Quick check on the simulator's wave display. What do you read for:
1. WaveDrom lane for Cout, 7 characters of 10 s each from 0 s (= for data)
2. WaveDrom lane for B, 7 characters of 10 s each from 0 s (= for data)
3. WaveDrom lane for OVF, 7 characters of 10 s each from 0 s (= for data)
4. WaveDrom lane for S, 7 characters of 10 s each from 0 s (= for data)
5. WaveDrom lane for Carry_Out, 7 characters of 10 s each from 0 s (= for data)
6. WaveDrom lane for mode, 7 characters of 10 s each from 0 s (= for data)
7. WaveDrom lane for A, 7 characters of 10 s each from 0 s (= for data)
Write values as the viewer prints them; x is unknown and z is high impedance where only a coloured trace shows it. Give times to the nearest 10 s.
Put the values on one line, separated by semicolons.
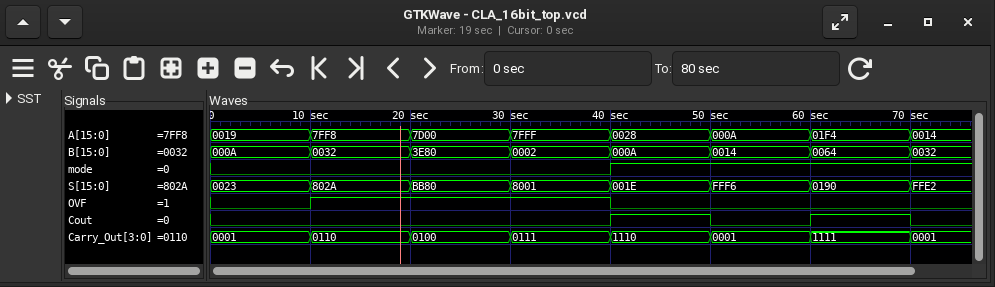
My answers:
{name: 'Cout', wave: '0...101'}; {name: 'B', wave: '=======', data: '000A 0032 3E80 0002 000A 0014 0064'}; {name: 'OVF', wave: '01..0..'}; {name: 'S', wave: '=======', data: '0023 802A BB80 8001 001E FFF6 0190'}; {name: 'Carry_Out', wave: '=======', data: '0001 0110 0100 0111 1110 0001 1111'}; {name: 'mode', wave: '0...1..'}; {name: 'A', wave: '=======', data: '0019 7FF8 7D00 7FFF 0028 000A 01F4'}
